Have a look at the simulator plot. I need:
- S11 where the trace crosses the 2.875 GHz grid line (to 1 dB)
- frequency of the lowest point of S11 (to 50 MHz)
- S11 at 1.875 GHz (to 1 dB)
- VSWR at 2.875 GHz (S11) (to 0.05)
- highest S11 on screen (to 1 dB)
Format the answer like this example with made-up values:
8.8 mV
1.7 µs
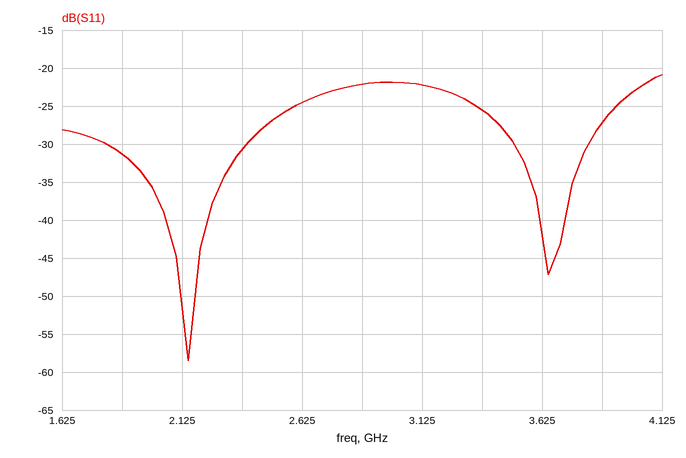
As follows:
-22 dB
2.15 GHz
-31 dB
1.15
-21 dB
